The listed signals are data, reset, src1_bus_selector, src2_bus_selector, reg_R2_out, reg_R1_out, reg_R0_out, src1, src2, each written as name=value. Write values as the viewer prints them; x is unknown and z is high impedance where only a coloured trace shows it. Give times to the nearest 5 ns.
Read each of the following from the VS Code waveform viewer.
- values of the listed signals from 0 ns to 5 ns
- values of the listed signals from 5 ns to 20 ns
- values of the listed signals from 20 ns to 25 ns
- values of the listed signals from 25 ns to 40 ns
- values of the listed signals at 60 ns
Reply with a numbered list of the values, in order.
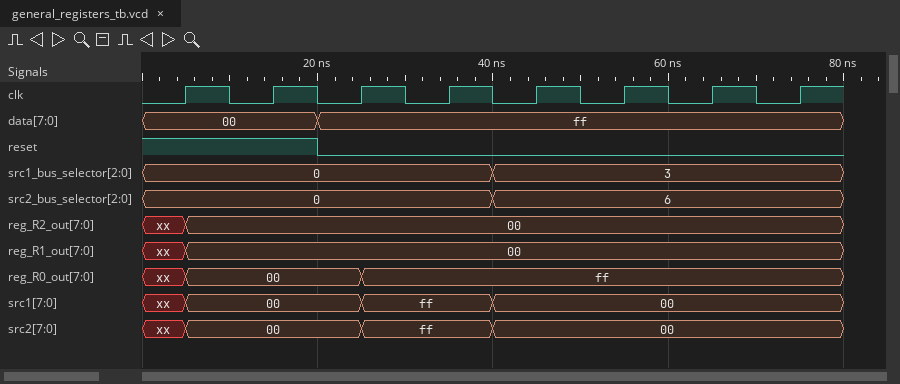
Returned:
1. data=00, reset=1, src1_bus_selector=0, src2_bus_selector=0, reg_R2_out=xx, reg_R1_out=xx, reg_R0_out=xx, src1=xx, src2=xx
2. data=00, reset=1, src1_bus_selector=0, src2_bus_selector=0, reg_R2_out=00, reg_R1_out=00, reg_R0_out=00, src1=00, src2=00
3. data=ff, reset=0, src1_bus_selector=0, src2_bus_selector=0, reg_R2_out=00, reg_R1_out=00, reg_R0_out=00, src1=00, src2=00
4. data=ff, reset=0, src1_bus_selector=0, src2_bus_selector=0, reg_R2_out=00, reg_R1_out=00, reg_R0_out=ff, src1=ff, src2=ff
5. data=ff, reset=0, src1_bus_selector=3, src2_bus_selector=6, reg_R2_out=00, reg_R1_out=00, reg_R0_out=ff, src1=00, src2=00
